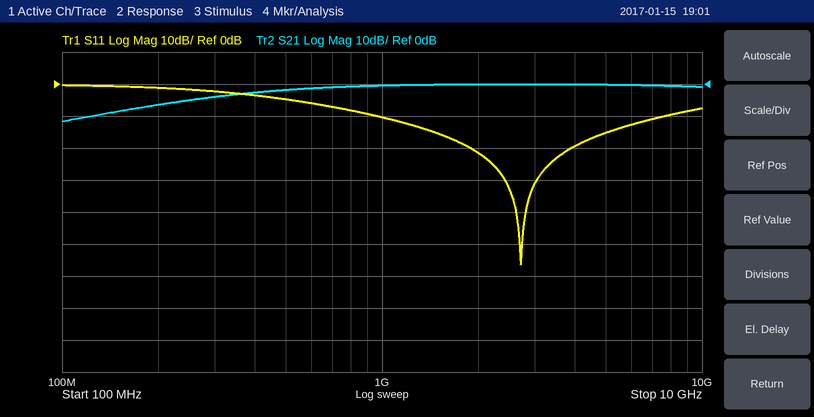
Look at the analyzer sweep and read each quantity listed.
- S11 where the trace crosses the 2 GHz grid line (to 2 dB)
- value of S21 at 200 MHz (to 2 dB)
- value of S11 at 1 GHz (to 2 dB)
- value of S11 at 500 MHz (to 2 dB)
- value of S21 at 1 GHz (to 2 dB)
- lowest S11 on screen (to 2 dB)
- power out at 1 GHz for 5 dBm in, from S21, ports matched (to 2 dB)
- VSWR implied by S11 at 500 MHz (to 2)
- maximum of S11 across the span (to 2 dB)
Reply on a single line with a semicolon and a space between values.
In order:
-22 dB; -6 dB; -10 dB; -4 dB; 0 dB; -56 dB; 4 dBm; 4; 0 dB
